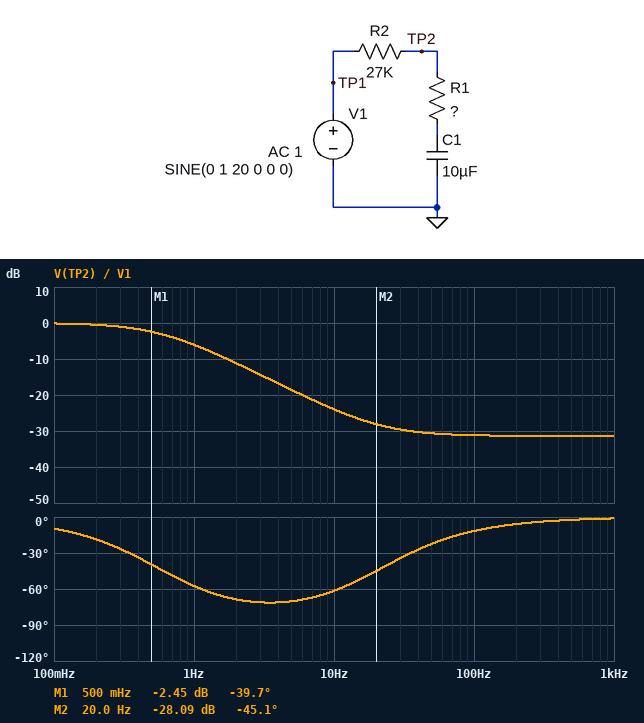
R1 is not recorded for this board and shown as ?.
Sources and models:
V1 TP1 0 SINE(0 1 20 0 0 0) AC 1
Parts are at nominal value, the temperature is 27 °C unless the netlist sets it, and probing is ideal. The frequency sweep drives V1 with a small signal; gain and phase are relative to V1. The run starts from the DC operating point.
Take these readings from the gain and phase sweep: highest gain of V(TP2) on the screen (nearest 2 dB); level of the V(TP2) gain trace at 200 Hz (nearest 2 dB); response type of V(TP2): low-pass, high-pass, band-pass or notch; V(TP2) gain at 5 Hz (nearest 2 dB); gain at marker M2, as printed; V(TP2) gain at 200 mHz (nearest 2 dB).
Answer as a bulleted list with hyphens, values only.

- 0 dB
- -32 dB
- low-pass
- -18 dB
- -28.09 dB
- 0 dB
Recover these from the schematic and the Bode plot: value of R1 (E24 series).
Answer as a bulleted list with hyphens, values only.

- 750 Ω
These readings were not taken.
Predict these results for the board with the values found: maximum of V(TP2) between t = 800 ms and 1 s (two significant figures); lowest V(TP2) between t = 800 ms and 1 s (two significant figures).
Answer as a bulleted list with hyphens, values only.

- 41 mV
- -39 mV
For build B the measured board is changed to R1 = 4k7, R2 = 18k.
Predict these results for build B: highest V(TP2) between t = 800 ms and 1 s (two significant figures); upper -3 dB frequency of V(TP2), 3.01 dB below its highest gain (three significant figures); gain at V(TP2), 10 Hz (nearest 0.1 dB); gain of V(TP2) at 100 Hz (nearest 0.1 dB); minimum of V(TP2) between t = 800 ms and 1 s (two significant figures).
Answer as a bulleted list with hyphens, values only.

- 210 mV
- 733 mHz
- -13.2 dB
- -13.7 dB
- -210 mV
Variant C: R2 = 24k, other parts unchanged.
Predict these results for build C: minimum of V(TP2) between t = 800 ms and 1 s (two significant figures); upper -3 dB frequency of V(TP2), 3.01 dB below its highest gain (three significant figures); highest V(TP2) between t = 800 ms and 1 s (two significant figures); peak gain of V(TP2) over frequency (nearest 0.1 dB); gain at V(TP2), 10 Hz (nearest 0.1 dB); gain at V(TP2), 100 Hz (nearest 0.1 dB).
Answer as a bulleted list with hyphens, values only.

- -44 mV
- 644 mHz
- 45 mV
- 0 dB
- -23.0 dB
- -30.2 dB
